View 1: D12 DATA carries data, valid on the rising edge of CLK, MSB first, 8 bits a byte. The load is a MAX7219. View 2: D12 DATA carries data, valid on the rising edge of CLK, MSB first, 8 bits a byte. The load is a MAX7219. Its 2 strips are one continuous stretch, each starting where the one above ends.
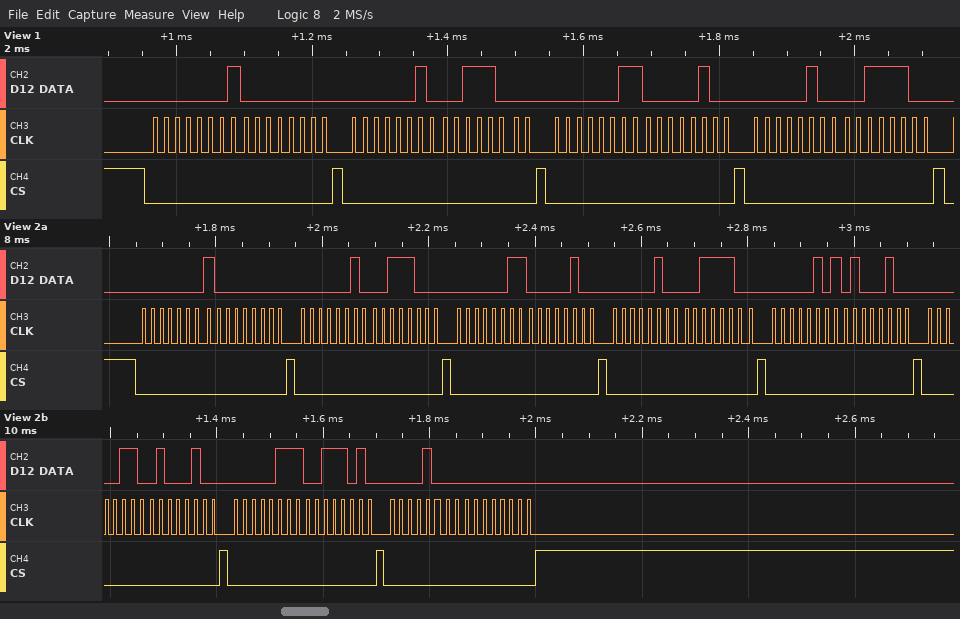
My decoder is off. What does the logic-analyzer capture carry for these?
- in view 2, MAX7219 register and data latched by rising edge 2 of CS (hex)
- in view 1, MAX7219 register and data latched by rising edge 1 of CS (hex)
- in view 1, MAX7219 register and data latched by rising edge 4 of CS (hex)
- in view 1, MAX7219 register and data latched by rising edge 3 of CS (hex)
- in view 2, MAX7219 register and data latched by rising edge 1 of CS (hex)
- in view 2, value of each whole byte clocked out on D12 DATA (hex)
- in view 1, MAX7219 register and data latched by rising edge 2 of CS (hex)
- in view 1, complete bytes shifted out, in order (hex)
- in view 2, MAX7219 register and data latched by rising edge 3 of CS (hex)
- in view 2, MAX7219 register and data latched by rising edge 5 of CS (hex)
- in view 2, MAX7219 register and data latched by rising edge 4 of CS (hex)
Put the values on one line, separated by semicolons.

register 0x2, data 0x38; register 0x1, data 0x00; register 0x4, data 0x3C; register 0x3, data 0x04; register 0x1, data 0x00; 01 00 02 38 03 04 04 3C 05 44 06 44 07 3A 08 00; register 0x2, data 0x38; 01 00 02 38 03 04 04 3C; register 0x3, data 0x04; register 0x5, data 0x44; register 0x4, data 0x3C
